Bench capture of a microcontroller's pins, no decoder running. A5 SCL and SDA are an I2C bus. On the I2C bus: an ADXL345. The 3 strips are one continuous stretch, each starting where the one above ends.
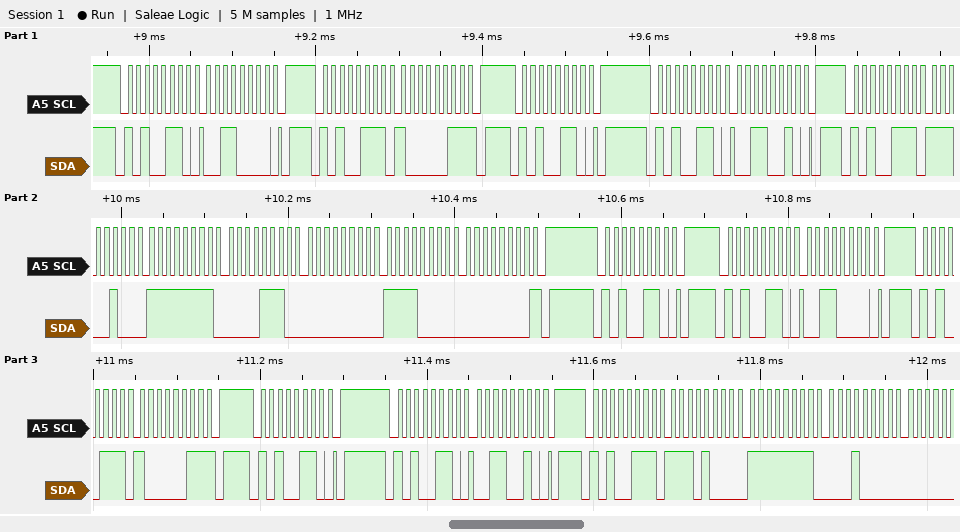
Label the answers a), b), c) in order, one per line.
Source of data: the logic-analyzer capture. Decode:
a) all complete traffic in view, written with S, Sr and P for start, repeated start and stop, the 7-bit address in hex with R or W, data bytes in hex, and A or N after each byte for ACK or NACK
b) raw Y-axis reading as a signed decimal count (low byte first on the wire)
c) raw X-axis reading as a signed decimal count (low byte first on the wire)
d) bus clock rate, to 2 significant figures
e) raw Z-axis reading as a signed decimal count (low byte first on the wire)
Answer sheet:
a) S 53W A 30 A P S 53R A 83 N P S 53W A P S 53W A 32 A P S 53R A E4 A FF A 0E A 00 A F0 A 00 N P S 53W A P S 53W A 30 A P S 53R A 83 N P S 53W A P S 53W A 32 A P S 53R A E8 A FF A 10 A
b) 14
c) -28
d) 100 kHz
e) 240
